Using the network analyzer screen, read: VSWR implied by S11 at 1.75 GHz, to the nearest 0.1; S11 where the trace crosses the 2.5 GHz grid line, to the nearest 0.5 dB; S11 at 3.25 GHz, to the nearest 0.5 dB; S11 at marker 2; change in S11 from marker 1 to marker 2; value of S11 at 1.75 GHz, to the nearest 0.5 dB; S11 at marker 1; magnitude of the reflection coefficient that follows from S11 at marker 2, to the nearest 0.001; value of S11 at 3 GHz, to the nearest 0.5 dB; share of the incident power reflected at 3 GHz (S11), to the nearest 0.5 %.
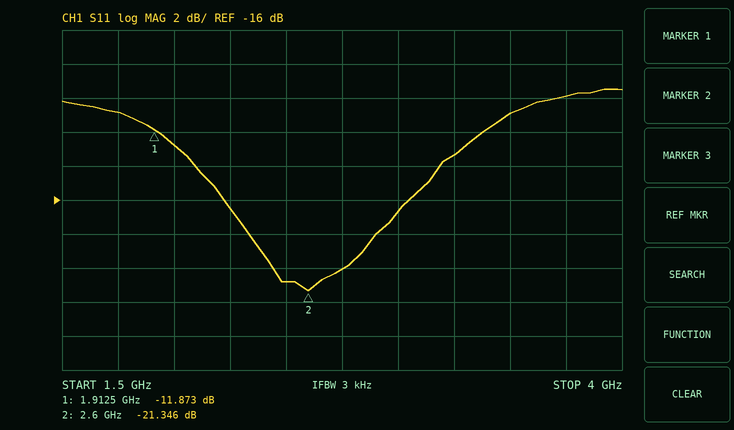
1.8
-21.0 dB
-13.5 dB
-21.346 dB
-9.473 dB
-11.0 dB
-11.873 dB
0.086
-16.5 dB
2.0 %
